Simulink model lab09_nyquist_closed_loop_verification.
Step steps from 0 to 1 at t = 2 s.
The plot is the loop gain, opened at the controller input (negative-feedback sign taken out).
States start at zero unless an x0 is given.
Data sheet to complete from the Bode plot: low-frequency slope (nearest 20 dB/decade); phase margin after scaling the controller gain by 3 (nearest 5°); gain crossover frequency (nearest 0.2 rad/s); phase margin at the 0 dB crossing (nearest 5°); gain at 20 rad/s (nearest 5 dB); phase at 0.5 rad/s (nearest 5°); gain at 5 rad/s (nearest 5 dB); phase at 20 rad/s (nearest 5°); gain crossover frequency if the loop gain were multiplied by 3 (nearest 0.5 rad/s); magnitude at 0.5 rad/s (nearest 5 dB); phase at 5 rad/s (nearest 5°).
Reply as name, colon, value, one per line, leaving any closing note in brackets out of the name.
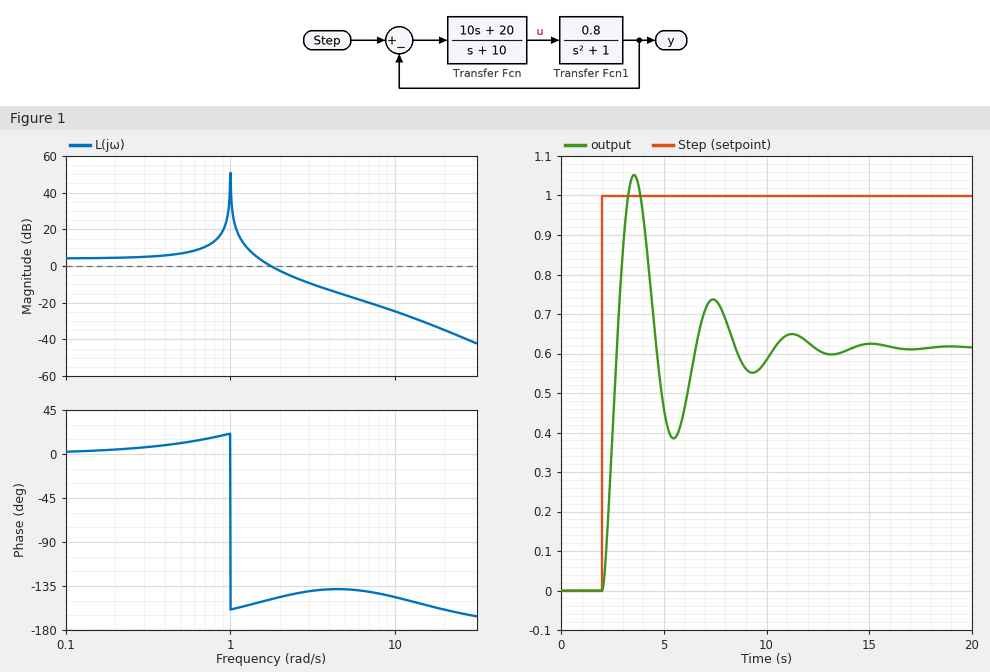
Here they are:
low-frequency slope: 0 dB/decade
phase margin after scaling the controller gain by 3: 40°
gain crossover frequency: 1.8 rad/s
phase margin at the 0 dB crossing: 30°
gain at 20 rad/s: -35 dB
phase at 0.5 rad/s: 10°
gain at 5 rad/s: -15 dB
phase at 20 rad/s: -160°
gain crossover frequency if the loop gain were multiplied by 3: 3.0 rad/s
magnitude at 0.5 rad/s: 5 dB
phase at 5 rad/s: -140°
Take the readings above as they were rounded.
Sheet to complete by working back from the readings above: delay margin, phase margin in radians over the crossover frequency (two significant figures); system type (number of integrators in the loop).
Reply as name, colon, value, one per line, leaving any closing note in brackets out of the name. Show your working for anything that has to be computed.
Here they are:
delay margin, phase margin in radians over the crossover frequency: 30 × π / 180 / 1.8 = 0.29 s
system type: 0
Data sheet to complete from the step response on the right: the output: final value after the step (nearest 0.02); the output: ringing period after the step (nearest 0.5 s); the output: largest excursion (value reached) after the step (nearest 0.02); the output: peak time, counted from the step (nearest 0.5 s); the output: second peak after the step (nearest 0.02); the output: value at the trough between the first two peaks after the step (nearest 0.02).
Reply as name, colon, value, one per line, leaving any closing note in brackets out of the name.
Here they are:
the output: final value after the step: 0.62
the output: ringing period after the step: 4.0 s
the output: largest excursion (value reached) after the step: 1.06
the output: peak time, counted from the step: 1.5 s
the output: second peak after the step: 0.74
the output: value at the trough between the first two peaks after the step: 0.38
